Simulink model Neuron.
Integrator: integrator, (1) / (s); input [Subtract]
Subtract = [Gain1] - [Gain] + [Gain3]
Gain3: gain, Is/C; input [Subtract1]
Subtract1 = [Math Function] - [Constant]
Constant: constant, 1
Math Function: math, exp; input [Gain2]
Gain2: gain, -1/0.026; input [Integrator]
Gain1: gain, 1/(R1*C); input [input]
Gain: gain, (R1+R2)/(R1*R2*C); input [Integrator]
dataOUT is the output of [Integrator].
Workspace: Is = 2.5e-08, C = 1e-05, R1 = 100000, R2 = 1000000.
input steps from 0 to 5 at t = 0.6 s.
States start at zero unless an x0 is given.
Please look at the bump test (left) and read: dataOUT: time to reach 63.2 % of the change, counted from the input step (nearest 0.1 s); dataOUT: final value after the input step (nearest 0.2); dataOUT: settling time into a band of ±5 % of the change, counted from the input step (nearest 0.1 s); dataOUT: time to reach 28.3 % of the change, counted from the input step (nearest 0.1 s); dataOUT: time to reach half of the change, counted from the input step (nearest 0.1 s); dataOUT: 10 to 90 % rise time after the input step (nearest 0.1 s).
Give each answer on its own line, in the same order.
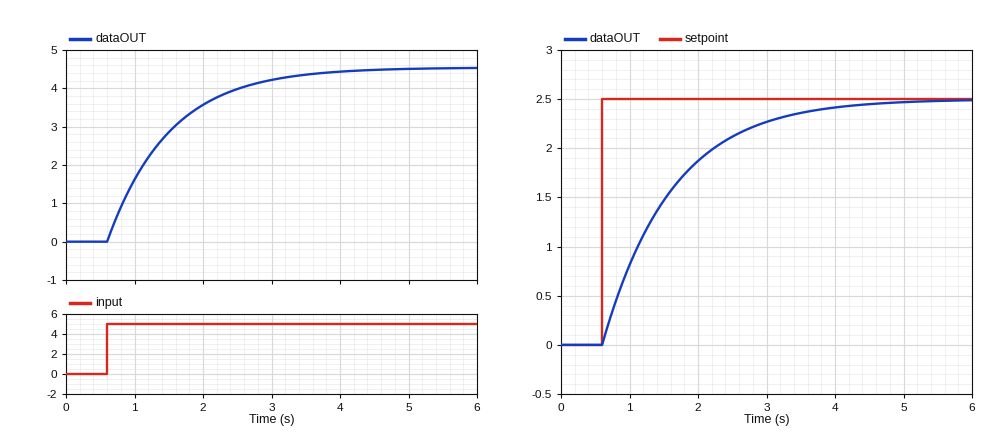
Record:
0.9 s
4.6
2.7 s
0.3 s
0.6 s
2.0 s
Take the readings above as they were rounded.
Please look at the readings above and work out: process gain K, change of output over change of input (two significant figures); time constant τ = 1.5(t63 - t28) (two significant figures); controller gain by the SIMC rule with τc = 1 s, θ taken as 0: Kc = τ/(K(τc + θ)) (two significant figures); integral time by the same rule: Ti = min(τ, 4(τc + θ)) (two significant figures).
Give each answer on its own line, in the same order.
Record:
0.92
0.90 s
0.98
0.90 s
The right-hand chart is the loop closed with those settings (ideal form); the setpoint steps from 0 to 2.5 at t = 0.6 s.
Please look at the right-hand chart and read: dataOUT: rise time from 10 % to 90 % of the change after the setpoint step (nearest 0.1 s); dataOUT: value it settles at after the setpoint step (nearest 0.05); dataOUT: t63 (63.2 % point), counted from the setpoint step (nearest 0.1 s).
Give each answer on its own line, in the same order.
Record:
2.2 s
2.50
1.0 s
